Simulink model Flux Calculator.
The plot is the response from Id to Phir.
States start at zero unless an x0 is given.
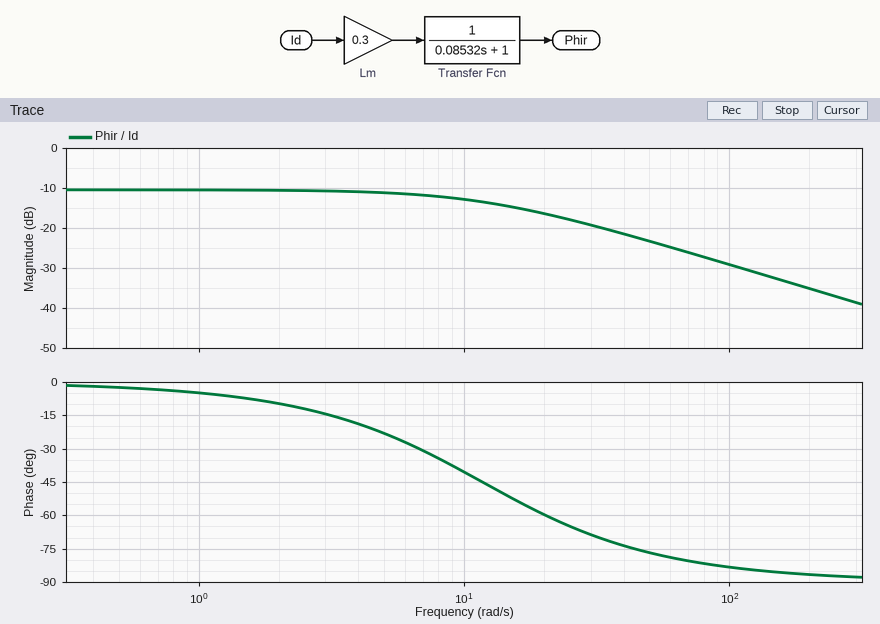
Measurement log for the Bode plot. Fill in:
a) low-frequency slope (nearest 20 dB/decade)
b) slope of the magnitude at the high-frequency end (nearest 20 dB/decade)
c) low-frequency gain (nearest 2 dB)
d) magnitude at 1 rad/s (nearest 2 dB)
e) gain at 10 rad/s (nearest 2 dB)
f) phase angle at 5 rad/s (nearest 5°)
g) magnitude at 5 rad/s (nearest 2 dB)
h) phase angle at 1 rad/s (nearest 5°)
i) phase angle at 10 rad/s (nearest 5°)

0 dB/decade
-20 dB/decade
-10 dB
-10 dB
-12 dB
-25°
-12 dB
-5°
-40°
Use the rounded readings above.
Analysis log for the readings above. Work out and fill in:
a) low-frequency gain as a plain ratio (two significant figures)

0.32
